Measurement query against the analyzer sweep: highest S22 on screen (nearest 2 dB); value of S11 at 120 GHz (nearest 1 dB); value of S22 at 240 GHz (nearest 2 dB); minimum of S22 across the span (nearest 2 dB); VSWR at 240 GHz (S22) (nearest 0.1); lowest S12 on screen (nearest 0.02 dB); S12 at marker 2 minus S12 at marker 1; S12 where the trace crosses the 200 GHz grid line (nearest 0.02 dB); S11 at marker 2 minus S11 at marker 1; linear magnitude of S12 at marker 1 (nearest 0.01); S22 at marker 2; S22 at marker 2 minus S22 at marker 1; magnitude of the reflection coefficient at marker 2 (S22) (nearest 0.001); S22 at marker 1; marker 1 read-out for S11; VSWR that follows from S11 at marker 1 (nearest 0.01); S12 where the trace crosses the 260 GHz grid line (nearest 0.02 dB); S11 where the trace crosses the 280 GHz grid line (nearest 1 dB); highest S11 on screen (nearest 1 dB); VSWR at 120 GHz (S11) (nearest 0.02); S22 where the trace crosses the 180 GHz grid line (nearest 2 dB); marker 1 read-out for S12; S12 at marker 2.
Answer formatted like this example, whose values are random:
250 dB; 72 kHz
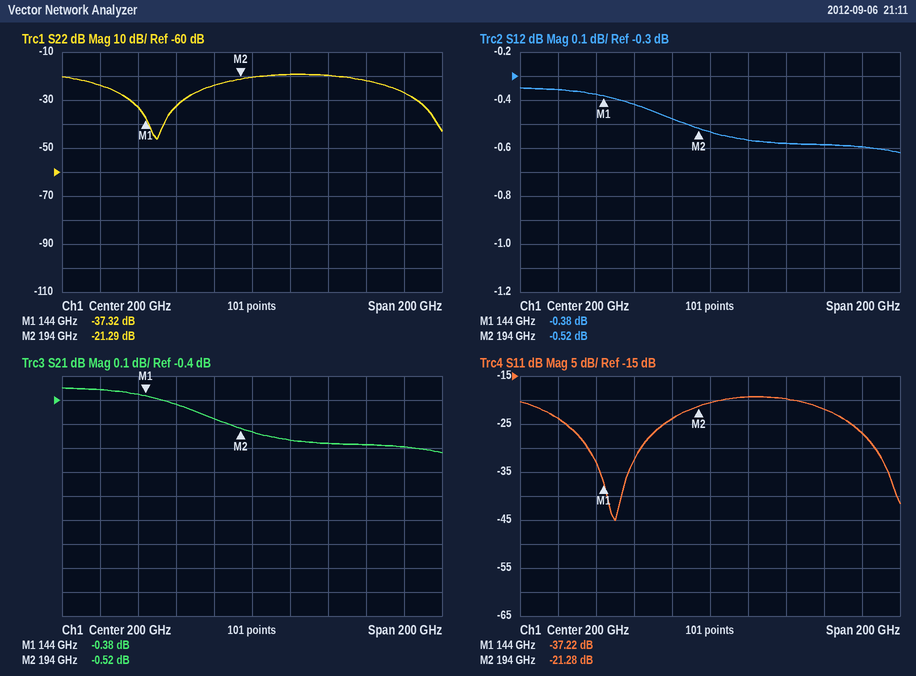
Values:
-20 dB; -24 dB; -20 dB; -46 dB; 1.2; -0.62 dB; -0.14 dB; -0.54 dB; 15.94 dB; 0.96; -21.29 dB; 16.03 dB; 0.086; -37.32 dB; -37.22 dB; 1.03; -0.58 dB; -27 dB; -19 dB; 1.14; -24 dB; -0.38 dB; -0.52 dB
